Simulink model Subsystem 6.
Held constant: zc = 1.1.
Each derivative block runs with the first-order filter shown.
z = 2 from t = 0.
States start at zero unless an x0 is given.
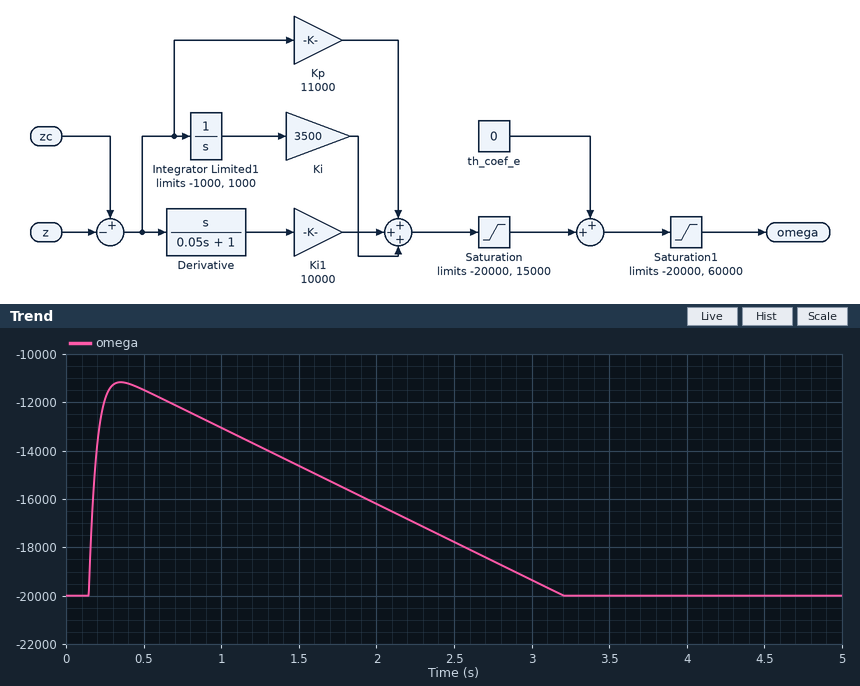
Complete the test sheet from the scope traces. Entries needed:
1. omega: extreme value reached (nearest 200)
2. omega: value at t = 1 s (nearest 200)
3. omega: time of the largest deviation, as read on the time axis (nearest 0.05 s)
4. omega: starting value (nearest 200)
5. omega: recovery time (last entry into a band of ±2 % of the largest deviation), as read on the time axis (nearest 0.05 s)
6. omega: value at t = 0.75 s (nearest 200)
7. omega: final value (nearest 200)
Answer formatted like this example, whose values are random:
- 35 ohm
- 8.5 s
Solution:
- -11200
- -13000
- 0.35 s
- -20000
- 3.15 s
- -12200
- -20000
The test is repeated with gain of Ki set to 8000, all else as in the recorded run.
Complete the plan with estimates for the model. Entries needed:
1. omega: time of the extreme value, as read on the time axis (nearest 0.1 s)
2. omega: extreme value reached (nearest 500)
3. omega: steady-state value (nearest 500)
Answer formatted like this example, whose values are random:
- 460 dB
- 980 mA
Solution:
- 0.3 s
- -12500
- -20000
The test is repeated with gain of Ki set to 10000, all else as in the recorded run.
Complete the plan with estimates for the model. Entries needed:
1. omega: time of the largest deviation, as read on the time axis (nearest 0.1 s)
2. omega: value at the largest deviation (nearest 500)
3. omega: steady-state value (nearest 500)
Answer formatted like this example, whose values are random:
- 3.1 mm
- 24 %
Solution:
- 0.3 s
- -13000
- -20000
